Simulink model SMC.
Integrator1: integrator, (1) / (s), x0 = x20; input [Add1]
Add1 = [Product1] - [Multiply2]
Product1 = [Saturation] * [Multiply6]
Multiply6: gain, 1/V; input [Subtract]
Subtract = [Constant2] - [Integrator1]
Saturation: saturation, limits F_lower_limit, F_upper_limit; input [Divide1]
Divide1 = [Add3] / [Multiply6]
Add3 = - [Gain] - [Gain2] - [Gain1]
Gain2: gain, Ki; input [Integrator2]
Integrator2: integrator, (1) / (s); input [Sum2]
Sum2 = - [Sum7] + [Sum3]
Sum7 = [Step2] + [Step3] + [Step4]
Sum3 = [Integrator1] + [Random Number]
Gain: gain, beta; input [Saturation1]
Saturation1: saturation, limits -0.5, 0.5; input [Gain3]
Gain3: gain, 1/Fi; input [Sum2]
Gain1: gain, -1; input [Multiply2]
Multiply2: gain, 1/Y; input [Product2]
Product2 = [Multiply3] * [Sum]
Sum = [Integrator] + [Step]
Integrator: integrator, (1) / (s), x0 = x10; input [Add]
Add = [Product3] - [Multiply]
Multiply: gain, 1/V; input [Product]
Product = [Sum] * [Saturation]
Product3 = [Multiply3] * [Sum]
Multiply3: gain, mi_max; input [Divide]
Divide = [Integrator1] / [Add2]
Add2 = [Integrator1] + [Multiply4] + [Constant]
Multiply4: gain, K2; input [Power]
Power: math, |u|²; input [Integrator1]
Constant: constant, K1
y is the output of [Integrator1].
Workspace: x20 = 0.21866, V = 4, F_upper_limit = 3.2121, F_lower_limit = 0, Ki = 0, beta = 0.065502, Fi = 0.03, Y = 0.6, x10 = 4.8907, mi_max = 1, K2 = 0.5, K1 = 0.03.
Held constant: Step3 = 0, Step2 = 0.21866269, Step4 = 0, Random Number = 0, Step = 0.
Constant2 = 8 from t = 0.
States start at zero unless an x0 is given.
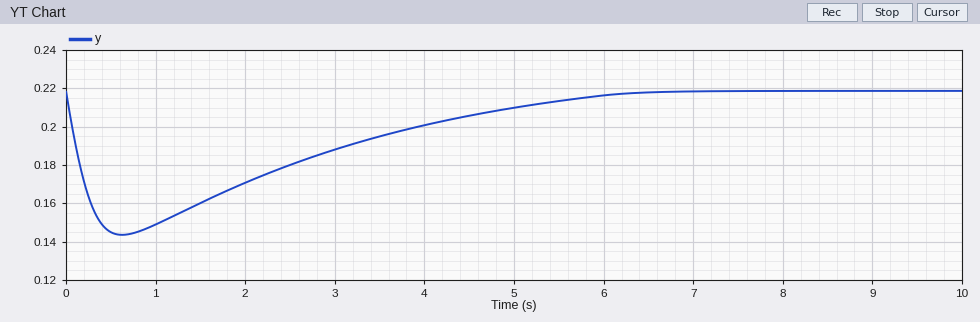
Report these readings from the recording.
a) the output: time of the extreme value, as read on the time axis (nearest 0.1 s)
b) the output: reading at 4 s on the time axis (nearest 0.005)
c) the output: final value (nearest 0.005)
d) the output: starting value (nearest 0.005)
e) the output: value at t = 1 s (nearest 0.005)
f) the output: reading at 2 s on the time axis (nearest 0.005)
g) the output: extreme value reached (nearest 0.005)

0.6 s
0.200
0.220
0.220
0.150
0.170
0.145
